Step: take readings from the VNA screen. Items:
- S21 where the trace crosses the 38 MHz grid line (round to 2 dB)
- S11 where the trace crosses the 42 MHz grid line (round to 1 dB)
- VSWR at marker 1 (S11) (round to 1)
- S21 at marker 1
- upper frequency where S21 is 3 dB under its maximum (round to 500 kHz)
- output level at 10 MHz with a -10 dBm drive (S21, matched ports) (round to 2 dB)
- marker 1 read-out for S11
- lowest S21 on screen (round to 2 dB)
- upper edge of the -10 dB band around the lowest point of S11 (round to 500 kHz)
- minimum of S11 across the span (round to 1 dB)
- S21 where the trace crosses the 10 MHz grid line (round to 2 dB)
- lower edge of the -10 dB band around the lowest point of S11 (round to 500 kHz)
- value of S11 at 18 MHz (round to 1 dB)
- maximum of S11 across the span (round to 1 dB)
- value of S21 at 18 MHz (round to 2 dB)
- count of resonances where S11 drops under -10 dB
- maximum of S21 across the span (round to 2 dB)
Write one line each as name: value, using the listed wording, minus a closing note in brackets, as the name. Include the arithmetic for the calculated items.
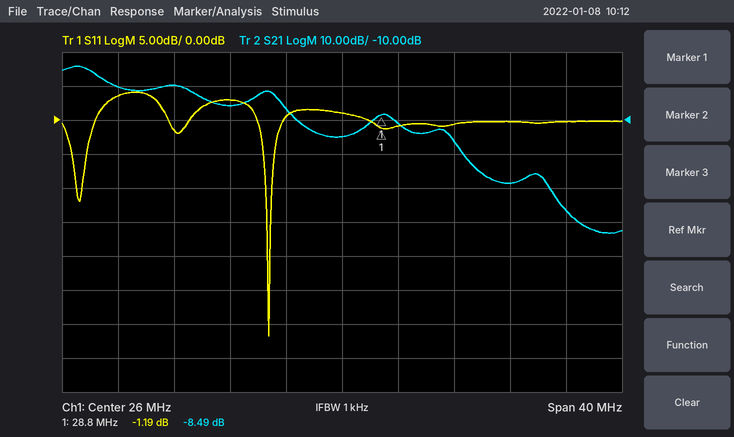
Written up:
S21 where the trace crosses the 38 MHz grid line: -28 dB
S11 where the trace crosses the 42 MHz grid line: 0 dB
VSWR at marker 1 (S11): (1 + 0.8720)/(1 − 0.8720) ≈ 15
S21 at marker 1: -8.49 dB
upper frequency where S21 is 3 dB under its maximum: 8.5 MHz
output level at 10 MHz with a -10 dBm drive (S21, matched ports): -10 dBm + (0 dB) = -10 dBm
marker 1 read-out for S11: -1.19 dB
lowest S21 on screen: -44 dB
upper edge of the -10 dB band around the lowest point of S11: 21.0 MHz
minimum of S11 across the span: -32 dB
S21 where the trace crosses the 10 MHz grid line: 0 dB
lower edge of the -10 dB band around the lowest point of S11: 20.5 MHz
value of S11 at 18 MHz: 3 dB
maximum of S11 across the span: 4 dB
value of S21 at 18 MHz: -6 dB
count of resonances where S11 drops under -10 dB: 2
maximum of S21 across the span: 6 dB
